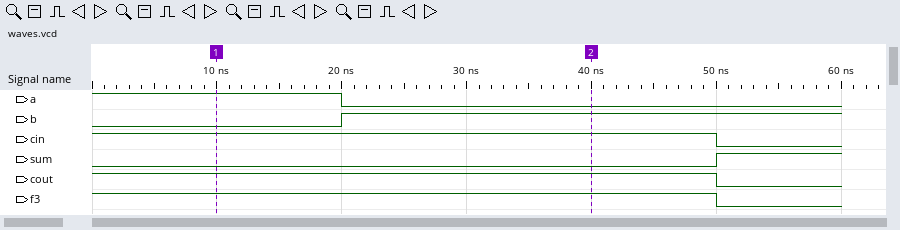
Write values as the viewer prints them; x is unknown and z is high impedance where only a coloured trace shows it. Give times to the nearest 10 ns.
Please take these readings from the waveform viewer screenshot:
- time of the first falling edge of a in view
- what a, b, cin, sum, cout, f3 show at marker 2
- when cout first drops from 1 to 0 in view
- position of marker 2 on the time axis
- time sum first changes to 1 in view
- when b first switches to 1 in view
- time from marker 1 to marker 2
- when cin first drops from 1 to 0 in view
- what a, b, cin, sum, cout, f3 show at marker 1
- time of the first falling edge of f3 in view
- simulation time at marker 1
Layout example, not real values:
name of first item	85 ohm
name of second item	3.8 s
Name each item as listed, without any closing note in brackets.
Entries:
time of the first falling edge of a in view	20 ns
what a, b, cin, sum, cout, f3 show at marker 2	a=0, b=1, cin=1, sum=0, cout=1, f3=1
when cout first drops from 1 to 0 in view	50 ns
position of marker 2 on the time axis	40 ns
time sum first changes to 1 in view	50 ns
when b first switches to 1 in view	20 ns
time from marker 1 to marker 2	30 ns
when cin first drops from 1 to 0 in view	50 ns
what a, b, cin, sum, cout, f3 show at marker 1	a=1, b=0, cin=1, sum=0, cout=1, f3=1
time of the first falling edge of f3 in view	50 ns
simulation time at marker 1	10 ns
